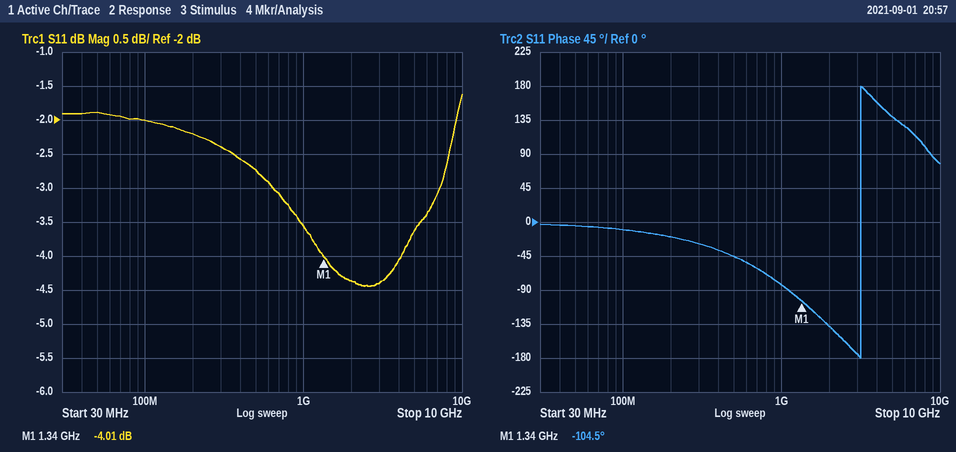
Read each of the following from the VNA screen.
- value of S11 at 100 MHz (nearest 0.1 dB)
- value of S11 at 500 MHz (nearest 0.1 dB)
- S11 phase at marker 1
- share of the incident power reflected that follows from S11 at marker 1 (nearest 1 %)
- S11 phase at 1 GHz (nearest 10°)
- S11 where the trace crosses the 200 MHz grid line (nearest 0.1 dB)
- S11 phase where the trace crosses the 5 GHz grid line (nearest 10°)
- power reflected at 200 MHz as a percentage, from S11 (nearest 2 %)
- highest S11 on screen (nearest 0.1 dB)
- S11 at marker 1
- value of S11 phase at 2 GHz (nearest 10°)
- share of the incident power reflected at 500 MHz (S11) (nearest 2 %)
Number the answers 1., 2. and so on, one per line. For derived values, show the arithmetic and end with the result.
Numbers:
1. -2.0 dB
2. -2.7 dB
3. -104.5°
4. 10^(-4.01/10) ≈ 40 %
5. -80°
6. -2.2 dB
7. 140°
8. 10^(-2.2/10) ≈ 60 %
9. -1.6 dB
10. -4.01 dB
11. -140°
12. 10^(-2.7/10) ≈ 54 %
